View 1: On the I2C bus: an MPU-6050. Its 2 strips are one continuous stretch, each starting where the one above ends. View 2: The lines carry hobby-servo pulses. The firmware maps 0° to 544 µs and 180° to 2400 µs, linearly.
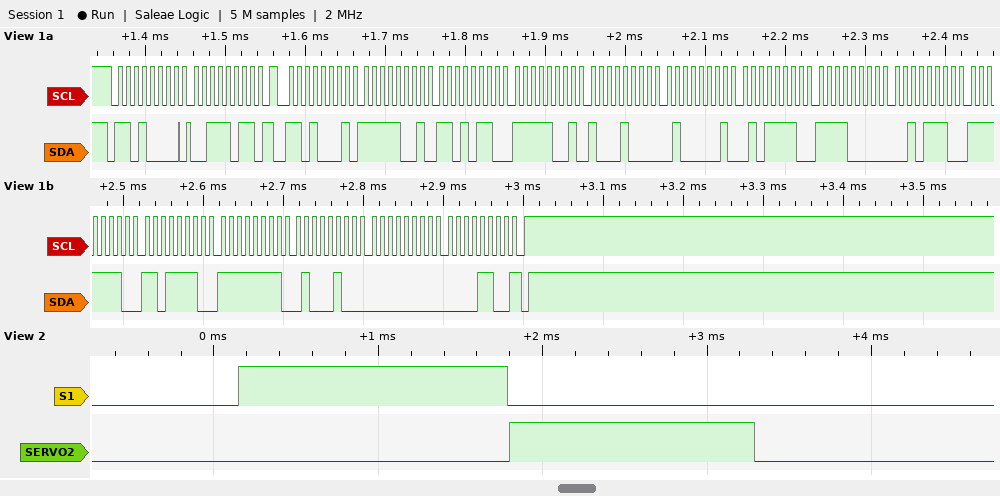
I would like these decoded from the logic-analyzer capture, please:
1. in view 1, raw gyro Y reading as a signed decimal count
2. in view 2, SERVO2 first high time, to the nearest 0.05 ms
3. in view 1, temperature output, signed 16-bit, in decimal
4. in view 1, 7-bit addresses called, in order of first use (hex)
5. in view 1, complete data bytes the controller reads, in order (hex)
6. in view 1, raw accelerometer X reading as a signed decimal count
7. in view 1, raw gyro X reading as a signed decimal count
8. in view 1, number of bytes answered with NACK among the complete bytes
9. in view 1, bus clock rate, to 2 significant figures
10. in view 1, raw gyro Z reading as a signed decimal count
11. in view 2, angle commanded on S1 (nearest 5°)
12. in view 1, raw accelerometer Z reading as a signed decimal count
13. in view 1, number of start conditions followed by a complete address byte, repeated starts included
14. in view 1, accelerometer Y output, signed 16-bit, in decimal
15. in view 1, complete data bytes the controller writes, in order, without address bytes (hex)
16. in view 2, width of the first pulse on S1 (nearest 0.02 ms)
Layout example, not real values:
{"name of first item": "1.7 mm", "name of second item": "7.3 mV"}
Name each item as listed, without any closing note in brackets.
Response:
{"in view 1, raw gyro Y reading as a signed decimal count": "-188", "in view 2, SERVO2 first high time, to the nearest 0.05 ms": "1.50 ms", "in view 1, temperature output, signed 16-bit, in decimal": "-4050", "in view 1, 7-bit addresses called, in order of first use": "0x68", "in view 1, complete data bytes the controller reads, in order": "F9 D6 F9 88 41 5E F0 2E FE DE FF 44 00 0C", "in view 1, raw accelerometer X reading as a signed decimal count": "-1578", "in view 1, raw gyro X reading as a signed decimal count": "-290", "in view 1, number of bytes answered with NACK among the complete bytes": "1", "in view 1, bus clock rate, to 2 significant figures": "100 kHz", "in view 1, raw gyro Z reading as a signed decimal count": "12", "in view 2, angle commanded on S1": "105°", "in view 1, raw accelerometer Z reading as a signed decimal count": "16734", "in view 1, number of start conditions followed by a complete address byte, repeated starts included": "2", "in view 1, accelerometer Y output, signed 16-bit, in decimal": "-1656", "in view 1, complete data bytes the controller writes, in order, without address bytes": "3B", "in view 2, width of the first pulse on S1": "1.64 ms"}
